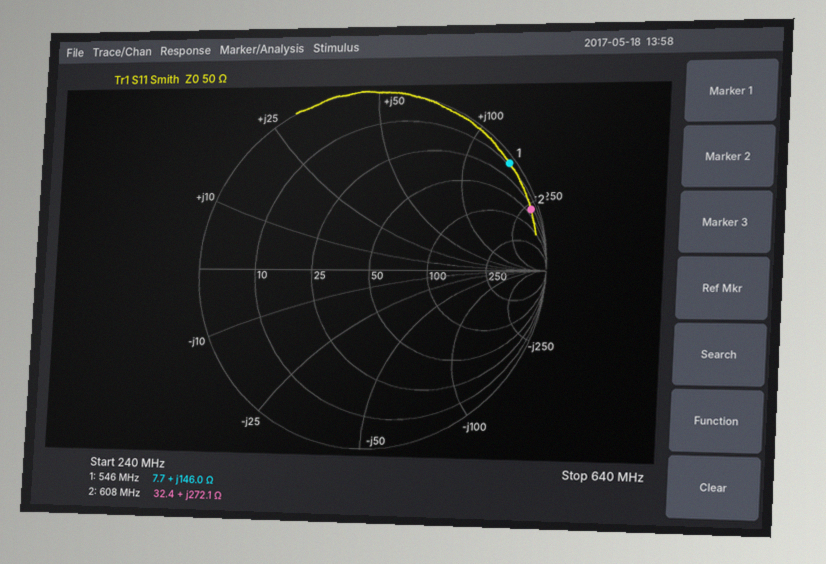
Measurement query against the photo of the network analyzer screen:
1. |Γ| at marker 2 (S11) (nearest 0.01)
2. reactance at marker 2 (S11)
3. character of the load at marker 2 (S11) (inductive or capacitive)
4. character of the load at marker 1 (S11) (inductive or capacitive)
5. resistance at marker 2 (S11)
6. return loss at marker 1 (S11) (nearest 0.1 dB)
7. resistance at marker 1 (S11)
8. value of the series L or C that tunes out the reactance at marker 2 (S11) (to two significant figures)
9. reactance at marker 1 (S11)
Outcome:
0.96
+272.1 Ω
inductive
inductive
32.4 Ω
0.3 dB
7.7 Ω
960 fF
+146.0 Ω
